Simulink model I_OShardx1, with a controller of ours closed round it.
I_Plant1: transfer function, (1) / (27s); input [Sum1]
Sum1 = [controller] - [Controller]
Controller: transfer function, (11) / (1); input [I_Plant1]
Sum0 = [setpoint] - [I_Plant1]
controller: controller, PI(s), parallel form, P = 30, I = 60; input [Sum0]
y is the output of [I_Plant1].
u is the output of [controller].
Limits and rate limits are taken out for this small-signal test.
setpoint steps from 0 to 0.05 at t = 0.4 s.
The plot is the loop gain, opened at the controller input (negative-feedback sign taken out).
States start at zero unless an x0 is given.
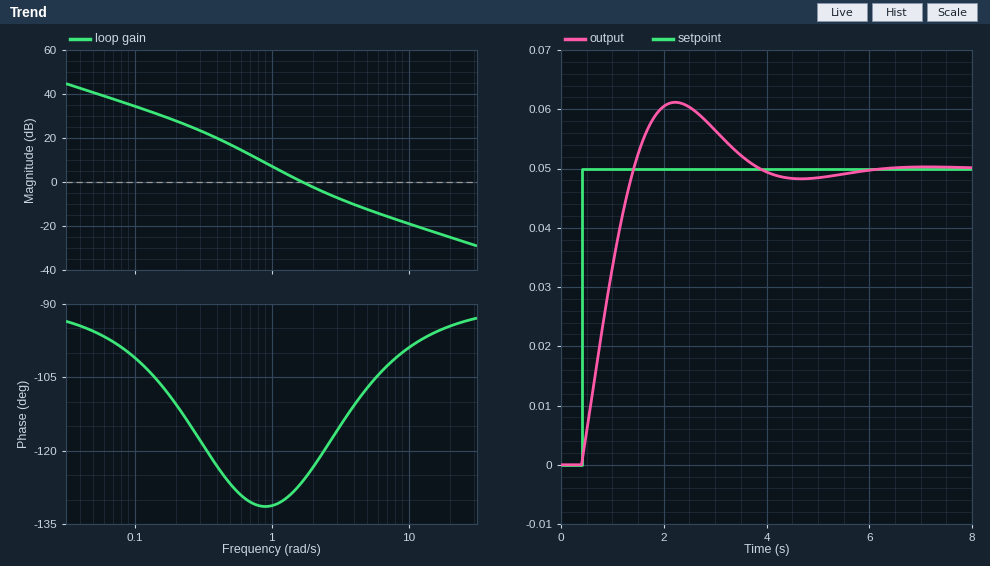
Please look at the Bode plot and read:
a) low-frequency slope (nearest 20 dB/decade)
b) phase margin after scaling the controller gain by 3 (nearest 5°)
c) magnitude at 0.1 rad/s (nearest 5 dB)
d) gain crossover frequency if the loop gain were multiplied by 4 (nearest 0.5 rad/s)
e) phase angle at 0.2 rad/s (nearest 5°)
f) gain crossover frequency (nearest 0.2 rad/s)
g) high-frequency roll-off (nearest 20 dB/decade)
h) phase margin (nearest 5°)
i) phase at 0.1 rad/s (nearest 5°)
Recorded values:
-20 dB/decade
70°
35 dB
5.0 rad/s
-110°
1.6 rad/s
-20 dB/decade
55°
-100°
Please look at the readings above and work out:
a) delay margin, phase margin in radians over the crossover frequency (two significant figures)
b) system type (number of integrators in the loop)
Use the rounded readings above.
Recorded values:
0.60 s
1
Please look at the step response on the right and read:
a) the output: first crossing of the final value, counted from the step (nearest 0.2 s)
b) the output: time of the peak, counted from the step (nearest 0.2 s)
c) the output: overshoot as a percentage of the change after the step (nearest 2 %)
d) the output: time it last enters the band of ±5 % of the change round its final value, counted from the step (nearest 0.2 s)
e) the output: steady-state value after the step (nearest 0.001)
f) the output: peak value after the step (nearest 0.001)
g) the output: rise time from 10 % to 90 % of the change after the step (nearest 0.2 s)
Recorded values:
1.0 s
1.8 s
22 %
3.0 s
0.050
0.061
0.8 s
